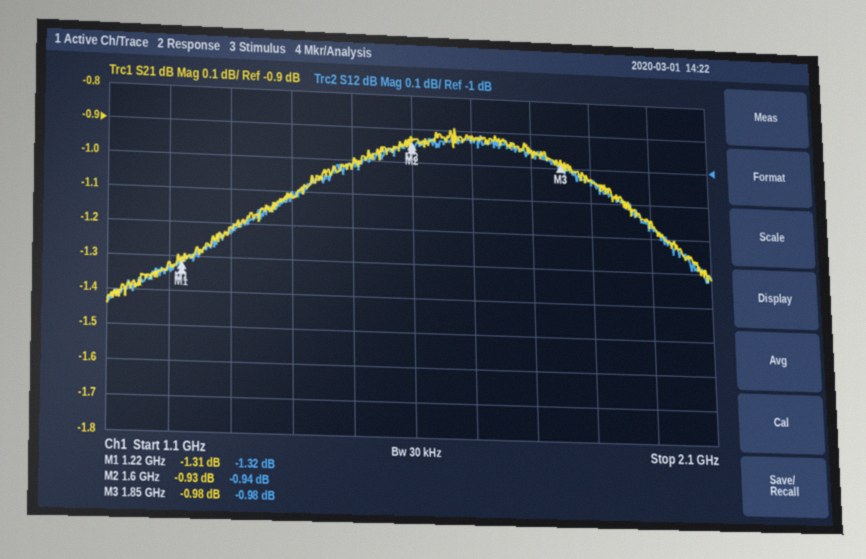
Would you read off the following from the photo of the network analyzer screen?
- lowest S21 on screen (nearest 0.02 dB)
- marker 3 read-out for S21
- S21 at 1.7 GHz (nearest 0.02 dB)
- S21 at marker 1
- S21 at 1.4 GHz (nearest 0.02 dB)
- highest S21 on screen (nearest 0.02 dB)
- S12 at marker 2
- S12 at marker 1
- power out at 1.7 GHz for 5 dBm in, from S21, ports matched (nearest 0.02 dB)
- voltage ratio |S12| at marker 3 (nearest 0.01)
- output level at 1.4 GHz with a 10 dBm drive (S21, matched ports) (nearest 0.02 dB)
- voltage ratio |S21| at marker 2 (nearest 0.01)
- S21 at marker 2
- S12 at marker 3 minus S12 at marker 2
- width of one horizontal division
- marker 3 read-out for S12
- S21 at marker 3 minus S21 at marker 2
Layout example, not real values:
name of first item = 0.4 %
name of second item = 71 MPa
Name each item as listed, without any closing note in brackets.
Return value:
lowest S21 on screen = -1.44 dB
marker 3 read-out for S21 = -0.98 dB
S21 at 1.7 GHz = -0.92 dB
S21 at marker 1 = -1.31 dB
S21 at 1.4 GHz = -1.12 dB
highest S21 on screen = -0.90 dB
S12 at marker 2 = -0.94 dB
S12 at marker 1 = -1.32 dB
power out at 1.7 GHz for 5 dBm in, from S21, ports matched = 4.08 dBm
voltage ratio |S12| at marker 3 = 0.89
output level at 1.4 GHz with a 10 dBm drive (S21, matched ports) = 8.88 dBm
voltage ratio |S21| at marker 2 = 0.90
S21 at marker 2 = -0.93 dB
S12 at marker 3 minus S12 at marker 2 = -0.04 dB
width of one horizontal division = 100 MHz
marker 3 read-out for S12 = -0.98 dB
S21 at marker 3 minus S21 at marker 2 = -0.05 dB
